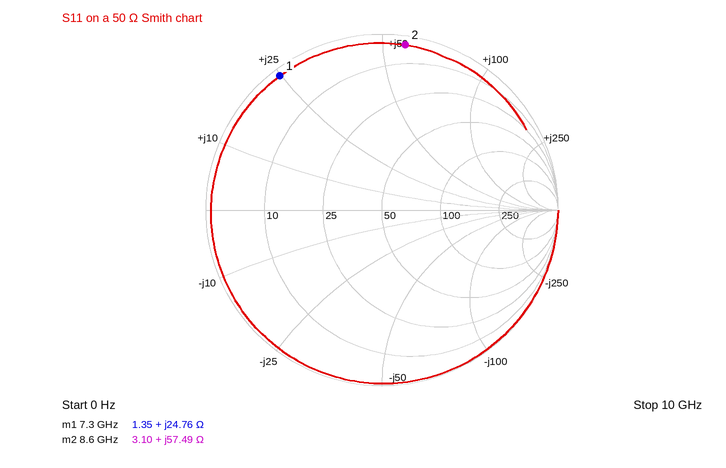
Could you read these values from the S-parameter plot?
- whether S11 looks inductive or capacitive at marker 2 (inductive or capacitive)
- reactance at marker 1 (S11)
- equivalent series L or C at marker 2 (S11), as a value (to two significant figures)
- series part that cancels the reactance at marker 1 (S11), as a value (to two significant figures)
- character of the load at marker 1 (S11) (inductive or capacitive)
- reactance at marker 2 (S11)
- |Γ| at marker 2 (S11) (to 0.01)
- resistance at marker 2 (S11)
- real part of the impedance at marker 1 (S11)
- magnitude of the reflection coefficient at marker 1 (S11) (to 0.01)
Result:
inductive
+24.76 Ω
1.1 nH
880 fF
inductive
+57.49 Ω
0.95
3.10 Ω
1.35 Ω
0.96
